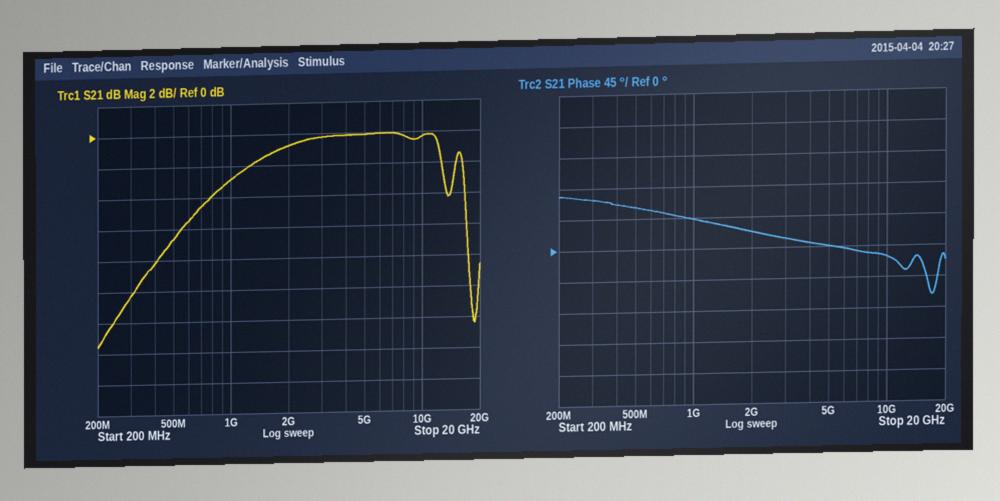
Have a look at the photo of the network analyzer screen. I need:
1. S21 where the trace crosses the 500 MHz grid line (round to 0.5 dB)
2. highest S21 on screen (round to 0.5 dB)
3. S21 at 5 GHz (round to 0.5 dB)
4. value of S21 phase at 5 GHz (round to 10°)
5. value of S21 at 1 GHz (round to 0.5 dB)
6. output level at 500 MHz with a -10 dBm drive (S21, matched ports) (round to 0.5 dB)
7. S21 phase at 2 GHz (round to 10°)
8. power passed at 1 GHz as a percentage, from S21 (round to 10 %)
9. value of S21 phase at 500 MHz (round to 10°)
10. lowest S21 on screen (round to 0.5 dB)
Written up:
-6.5 dB
0.0 dB
0.0 dB
0°
-3.0 dB
-16.5 dBm
20°
50 %
60°
-13.5 dB
